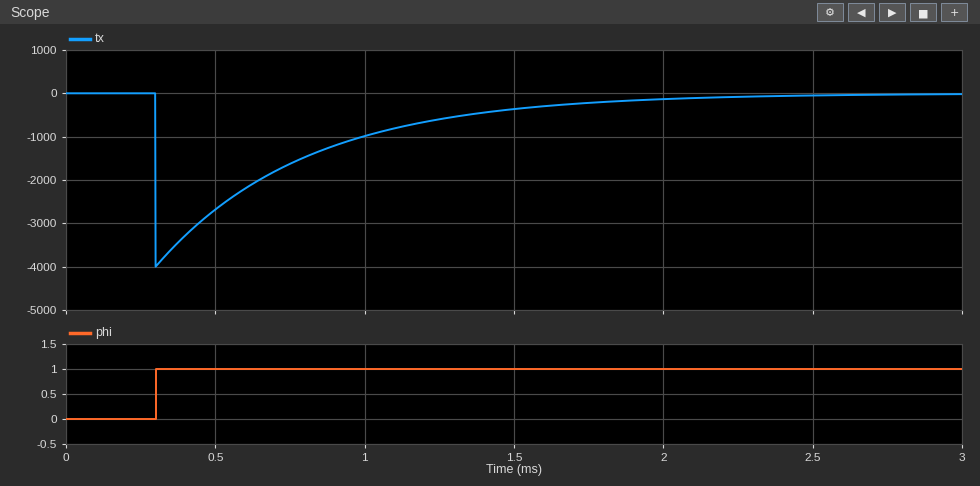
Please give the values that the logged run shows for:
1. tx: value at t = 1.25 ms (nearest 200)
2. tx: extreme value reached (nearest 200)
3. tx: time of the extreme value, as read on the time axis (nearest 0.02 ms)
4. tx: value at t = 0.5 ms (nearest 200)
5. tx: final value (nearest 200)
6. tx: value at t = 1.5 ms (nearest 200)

-600
-4000
0.30 ms
-2600
0
-400
